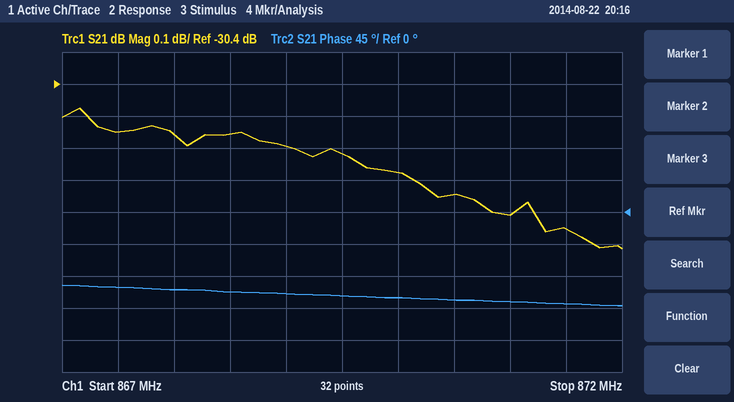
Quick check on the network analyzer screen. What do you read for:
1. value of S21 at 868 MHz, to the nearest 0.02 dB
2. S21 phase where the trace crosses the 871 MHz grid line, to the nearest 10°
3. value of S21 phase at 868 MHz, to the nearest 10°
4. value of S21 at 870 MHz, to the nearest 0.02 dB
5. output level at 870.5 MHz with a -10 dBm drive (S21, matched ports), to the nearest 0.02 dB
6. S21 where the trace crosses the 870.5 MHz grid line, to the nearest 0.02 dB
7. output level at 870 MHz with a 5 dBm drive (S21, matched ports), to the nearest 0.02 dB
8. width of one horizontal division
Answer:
-30.56 dB
-130°
-110°
-30.68 dB
-40.74 dBm
-30.74 dB
-25.68 dBm
500 kHz
